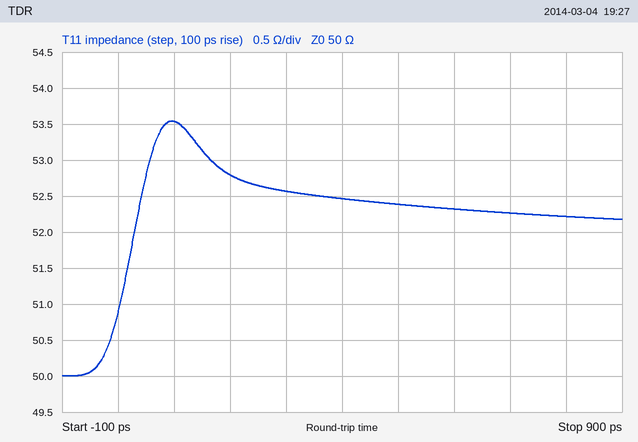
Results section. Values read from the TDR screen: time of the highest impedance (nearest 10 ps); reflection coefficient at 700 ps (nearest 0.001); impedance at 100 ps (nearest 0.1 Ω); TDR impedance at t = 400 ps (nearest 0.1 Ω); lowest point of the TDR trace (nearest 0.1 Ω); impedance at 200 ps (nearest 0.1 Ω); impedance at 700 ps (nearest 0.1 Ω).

100 ps
+0.022
53.5 Ω
52.5 Ω
50.0 Ω
52.8 Ω
52.3 Ω
